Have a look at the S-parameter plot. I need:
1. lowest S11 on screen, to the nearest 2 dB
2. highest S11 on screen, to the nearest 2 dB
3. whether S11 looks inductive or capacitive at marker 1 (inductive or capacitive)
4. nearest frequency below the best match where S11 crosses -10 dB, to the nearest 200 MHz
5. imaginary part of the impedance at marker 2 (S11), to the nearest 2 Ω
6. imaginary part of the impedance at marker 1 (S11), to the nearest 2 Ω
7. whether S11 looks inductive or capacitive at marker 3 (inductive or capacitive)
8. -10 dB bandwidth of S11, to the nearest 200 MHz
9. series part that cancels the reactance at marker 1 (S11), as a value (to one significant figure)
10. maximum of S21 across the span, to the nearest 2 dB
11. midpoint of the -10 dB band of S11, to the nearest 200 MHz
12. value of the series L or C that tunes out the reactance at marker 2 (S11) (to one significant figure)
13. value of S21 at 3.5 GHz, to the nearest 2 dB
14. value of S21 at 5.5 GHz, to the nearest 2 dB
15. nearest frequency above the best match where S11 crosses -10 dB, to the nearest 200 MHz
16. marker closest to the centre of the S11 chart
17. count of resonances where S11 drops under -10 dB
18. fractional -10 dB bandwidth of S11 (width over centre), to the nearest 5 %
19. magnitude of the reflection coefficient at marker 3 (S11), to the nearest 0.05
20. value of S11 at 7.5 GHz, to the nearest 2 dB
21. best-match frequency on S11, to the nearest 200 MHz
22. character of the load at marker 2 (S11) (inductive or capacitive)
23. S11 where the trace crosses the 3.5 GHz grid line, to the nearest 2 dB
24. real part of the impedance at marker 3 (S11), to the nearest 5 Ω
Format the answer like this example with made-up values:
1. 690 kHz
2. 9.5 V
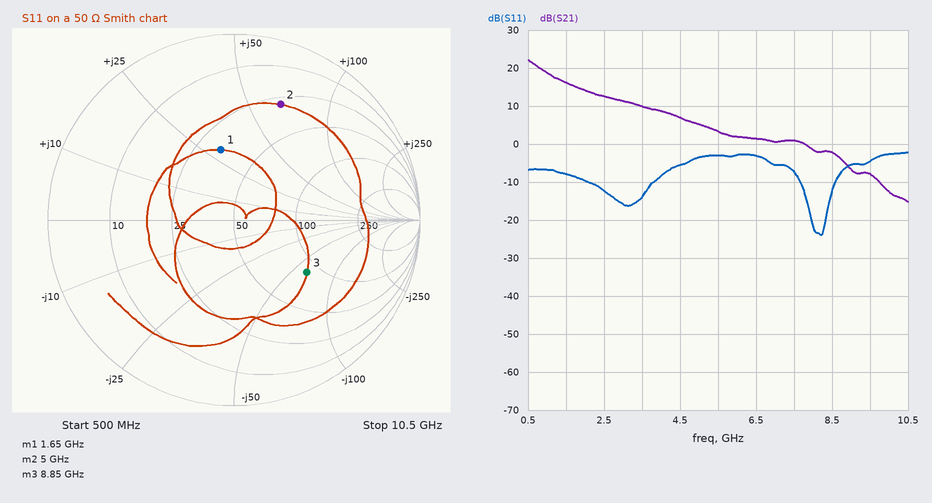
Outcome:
1. -24 dB
2. -2 dB
3. inductive
4. 7.6 GHz
5. +66 Ω
6. +30 Ω
7. capacitive
8. 1.0 GHz
9. 3 pF
10. 22 dB
11. 8.2 GHz
12. 500 fF
13. 10 dB
14. 4 dB
15. 8.6 GHz
16. marker 1
17. 2
18. 10 %
19. 0.50
20. -8 dB
21. 8.2 GHz
22. inductive
23. -14 dB
24. 85 Ω
